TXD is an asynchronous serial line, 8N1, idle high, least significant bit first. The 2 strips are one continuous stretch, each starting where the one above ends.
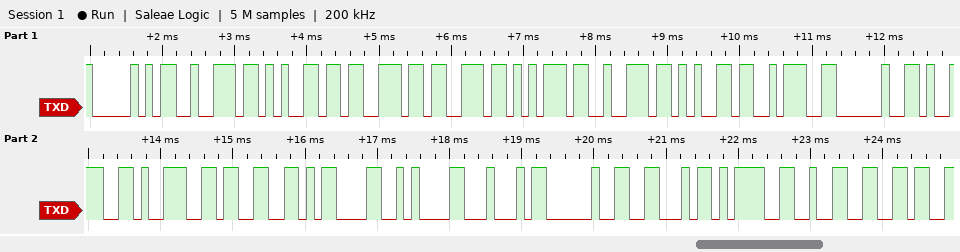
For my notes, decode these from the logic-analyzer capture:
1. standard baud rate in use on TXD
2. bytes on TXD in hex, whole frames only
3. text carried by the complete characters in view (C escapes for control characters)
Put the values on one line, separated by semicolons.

9600 baud; 50 72 65 73 73 75 72 65 3A 20 39 39 33 0D 0A 44 20 46 3D 32 36; "Pressure: 993\r\nD F=26"
